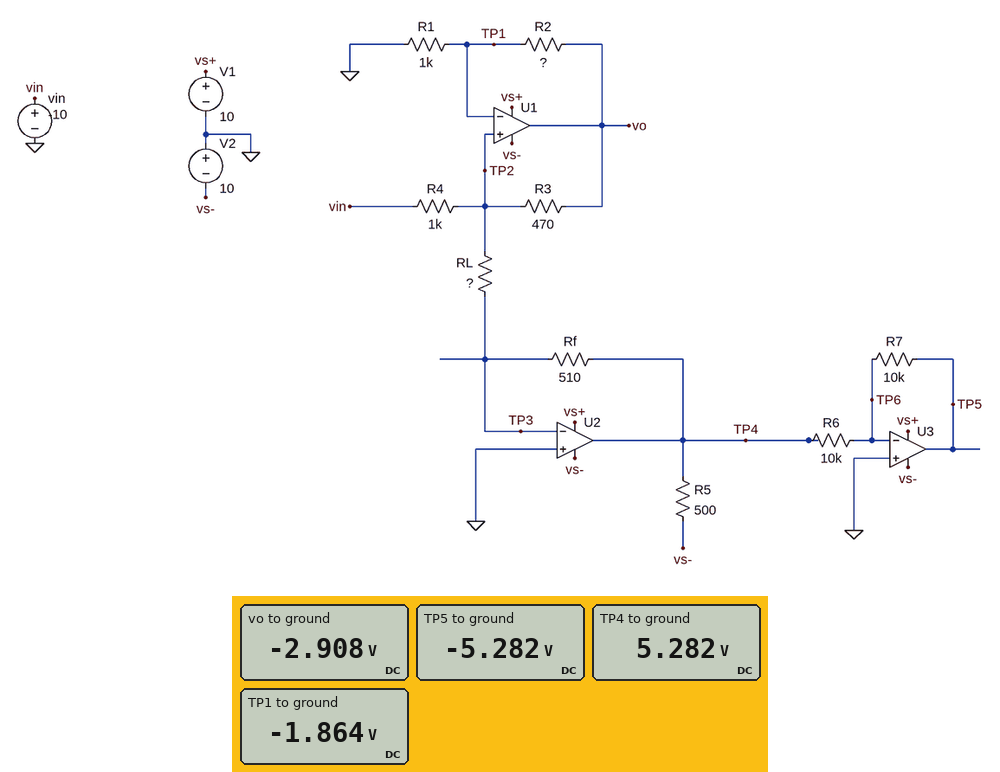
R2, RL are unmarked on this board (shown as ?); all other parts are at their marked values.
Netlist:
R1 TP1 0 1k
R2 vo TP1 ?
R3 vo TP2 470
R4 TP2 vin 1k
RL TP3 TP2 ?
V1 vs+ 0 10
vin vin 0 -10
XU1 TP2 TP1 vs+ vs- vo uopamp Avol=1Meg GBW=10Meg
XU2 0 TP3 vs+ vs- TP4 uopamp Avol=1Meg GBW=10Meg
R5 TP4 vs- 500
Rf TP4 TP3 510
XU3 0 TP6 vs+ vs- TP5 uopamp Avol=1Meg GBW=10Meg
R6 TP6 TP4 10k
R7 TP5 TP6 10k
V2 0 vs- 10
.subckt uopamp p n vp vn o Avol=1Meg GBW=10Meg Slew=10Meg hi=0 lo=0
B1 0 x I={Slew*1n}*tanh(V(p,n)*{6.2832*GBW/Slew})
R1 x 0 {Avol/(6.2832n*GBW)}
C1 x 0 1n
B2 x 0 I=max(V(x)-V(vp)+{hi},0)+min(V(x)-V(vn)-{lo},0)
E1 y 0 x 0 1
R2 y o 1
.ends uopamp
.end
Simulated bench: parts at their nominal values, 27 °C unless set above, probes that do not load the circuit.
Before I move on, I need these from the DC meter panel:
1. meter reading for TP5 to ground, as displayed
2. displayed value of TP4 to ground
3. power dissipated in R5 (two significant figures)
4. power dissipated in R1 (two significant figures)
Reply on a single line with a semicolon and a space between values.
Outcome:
-5.282 V; 5.282 V; 470 mW; 3.5 mW
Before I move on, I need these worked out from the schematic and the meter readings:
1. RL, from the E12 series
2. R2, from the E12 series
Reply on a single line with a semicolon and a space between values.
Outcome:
180 Ω; 560 Ω
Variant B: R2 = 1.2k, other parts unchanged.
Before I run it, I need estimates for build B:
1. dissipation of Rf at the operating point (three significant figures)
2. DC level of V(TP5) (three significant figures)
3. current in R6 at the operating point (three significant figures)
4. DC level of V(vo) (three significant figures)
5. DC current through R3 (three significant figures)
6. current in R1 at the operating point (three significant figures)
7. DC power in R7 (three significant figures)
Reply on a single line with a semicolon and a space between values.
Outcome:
98.3 mW; -7.08 V; 708 µA; -5.50 V; 6.38 mA; 2.50 mA; 5.01 mW
